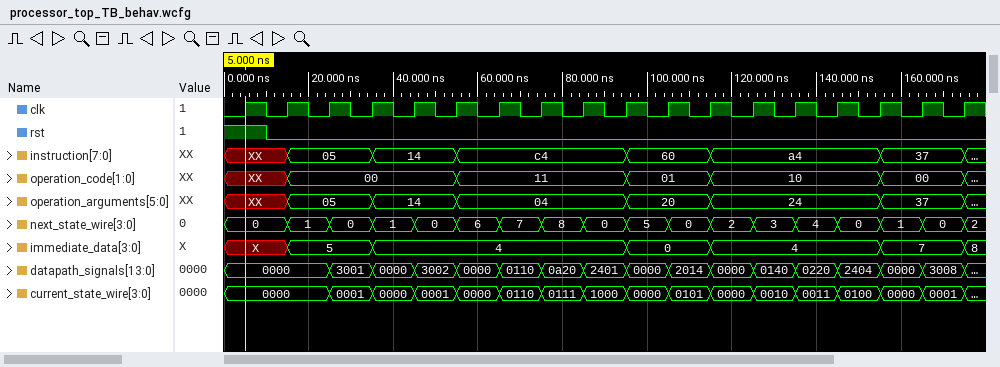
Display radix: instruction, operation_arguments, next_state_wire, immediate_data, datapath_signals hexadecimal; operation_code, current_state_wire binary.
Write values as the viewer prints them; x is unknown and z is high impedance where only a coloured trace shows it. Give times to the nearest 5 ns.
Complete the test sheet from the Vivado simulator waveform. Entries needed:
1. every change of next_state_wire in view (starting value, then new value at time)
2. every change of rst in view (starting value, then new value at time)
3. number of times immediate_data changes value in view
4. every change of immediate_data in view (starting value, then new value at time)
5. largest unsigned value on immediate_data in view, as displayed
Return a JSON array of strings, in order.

["0, 1 at 15 ns, 0 at 25 ns, 1 at 35 ns, 0 at 45 ns, 6 at 55 ns, 7 at 65 ns, 8 at 75 ns, 0 at 85 ns, 5 at 95 ns, 0 at 105 ns, 2 at 115 ns, 3 at 125 ns, 4 at 135 ns, 0 at 145 ns, 1 at 155 ns, 0 at 165 ns, 2 at 175 ns", "1, 0 at 10 ns", "6", "X, 5 at 15 ns, 4 at 35 ns, 0 at 95 ns, 4 at 115 ns, 7 at 155 ns, 8 at 175 ns", "8"]
